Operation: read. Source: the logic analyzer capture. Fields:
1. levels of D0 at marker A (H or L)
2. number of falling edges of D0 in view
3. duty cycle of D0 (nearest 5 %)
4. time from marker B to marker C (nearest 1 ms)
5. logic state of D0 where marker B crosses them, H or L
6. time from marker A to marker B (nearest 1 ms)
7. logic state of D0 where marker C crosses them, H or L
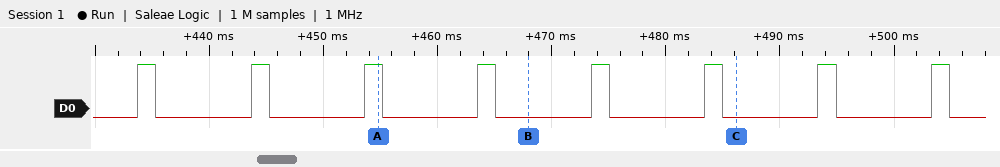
D0=H
8
15 %
18 ms
D0=L
13 ms
D0=L
